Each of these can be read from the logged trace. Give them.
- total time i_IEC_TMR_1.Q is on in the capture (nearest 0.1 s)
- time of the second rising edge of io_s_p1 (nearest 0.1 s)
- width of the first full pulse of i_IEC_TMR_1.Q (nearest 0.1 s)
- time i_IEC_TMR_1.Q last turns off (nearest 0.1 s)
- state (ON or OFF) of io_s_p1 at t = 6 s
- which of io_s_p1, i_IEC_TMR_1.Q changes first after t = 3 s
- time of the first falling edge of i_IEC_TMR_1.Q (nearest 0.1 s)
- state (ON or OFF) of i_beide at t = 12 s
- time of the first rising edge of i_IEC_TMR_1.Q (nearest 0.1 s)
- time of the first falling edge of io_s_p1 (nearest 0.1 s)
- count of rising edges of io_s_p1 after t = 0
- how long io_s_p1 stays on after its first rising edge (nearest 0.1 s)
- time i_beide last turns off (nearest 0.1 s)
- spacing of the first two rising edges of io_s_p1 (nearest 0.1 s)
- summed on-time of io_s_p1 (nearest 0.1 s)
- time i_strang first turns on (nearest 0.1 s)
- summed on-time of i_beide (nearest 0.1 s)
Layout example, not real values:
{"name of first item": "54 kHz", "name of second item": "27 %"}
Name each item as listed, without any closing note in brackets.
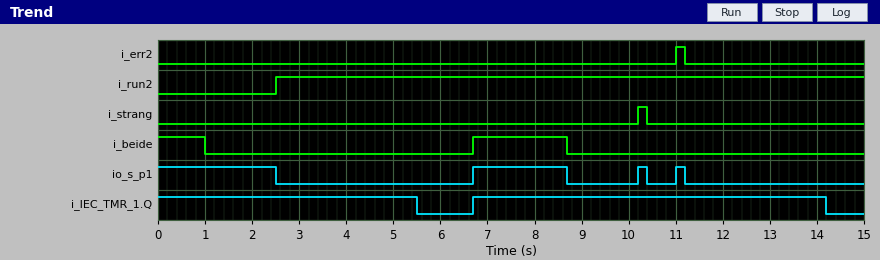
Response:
{"total time i_IEC_TMR_1.Q is on in the capture": "13.0 s", "time of the second rising edge of io_s_p1": "10.2 s", "width of the first full pulse of i_IEC_TMR_1.Q": "7.5 s", "time i_IEC_TMR_1.Q last turns off": "14.2 s", "state (ON or OFF) of io_s_p1 at t = 6 s": "OFF", "which of io_s_p1, i_IEC_TMR_1.Q changes first after t = 3 s": "i_IEC_TMR_1.Q", "time of the first falling edge of i_IEC_TMR_1.Q": "5.5 s", "state (ON or OFF) of i_beide at t = 12 s": "OFF", "time of the first rising edge of i_IEC_TMR_1.Q": "6.7 s", "time of the first falling edge of io_s_p1": "2.5 s", "count of rising edges of io_s_p1 after t = 0": "3", "how long io_s_p1 stays on after its first rising edge": "2.0 s", "time i_beide last turns off": "8.7 s", "spacing of the first two rising edges of io_s_p1": "3.5 s", "summed on-time of io_s_p1": "4.9 s", "time i_strang first turns on": "10.2 s", "summed on-time of i_beide": "3.0 s"}
